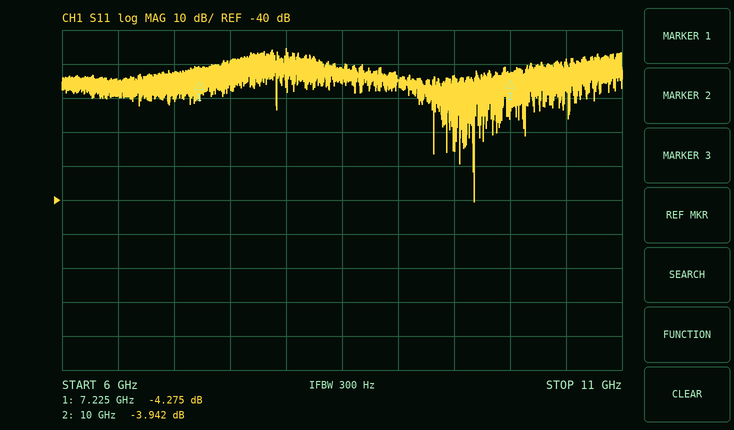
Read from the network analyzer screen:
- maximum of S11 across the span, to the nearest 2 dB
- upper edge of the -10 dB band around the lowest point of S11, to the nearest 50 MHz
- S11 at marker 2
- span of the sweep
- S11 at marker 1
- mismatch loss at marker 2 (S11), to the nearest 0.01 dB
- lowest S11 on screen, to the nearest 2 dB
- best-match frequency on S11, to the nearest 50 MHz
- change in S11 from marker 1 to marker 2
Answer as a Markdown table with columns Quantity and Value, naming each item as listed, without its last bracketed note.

| Quantity | Value |
|---|---|
| maximum of S11 across the span, to the nearest 2 dB | 4 dB |
| upper edge of the -10 dB band around the lowest point of S11, to the nearest 50 MHz | 9.70 GHz |
| S11 at marker 2 | -3.942 dB |
| span of the sweep | 5 GHz |
| S11 at marker 1 | -4.275 dB |
| mismatch loss at marker 2 (S11), to the nearest 0.01 dB | 2.24 dB |
| lowest S11 on screen, to the nearest 2 dB | -40 dB |
| best-match frequency on S11, to the nearest 50 MHz | 9.70 GHz |
| change in S11 from marker 1 to marker 2 | 0.333 dB |
